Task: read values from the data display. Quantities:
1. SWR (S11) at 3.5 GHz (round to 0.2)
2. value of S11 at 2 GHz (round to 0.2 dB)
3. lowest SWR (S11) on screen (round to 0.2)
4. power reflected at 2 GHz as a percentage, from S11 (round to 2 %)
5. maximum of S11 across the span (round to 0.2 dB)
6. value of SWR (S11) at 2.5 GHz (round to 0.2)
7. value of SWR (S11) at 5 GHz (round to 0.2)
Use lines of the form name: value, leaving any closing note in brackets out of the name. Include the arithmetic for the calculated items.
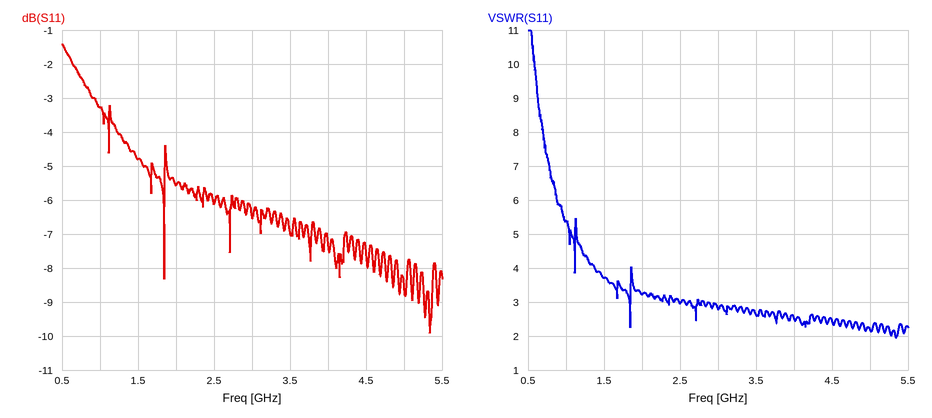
SWR (S11) at 3.5 GHz: 2.6
value of S11 at 2 GHz: -5.6 dB
lowest SWR (S11) on screen: 2.0
power reflected at 2 GHz as a percentage, from S11: 10^(-5.6/10) ≈ 28 %
maximum of S11 across the span: -1.4 dB
value of SWR (S11) at 2.5 GHz: 3.0
value of SWR (S11) at 5 GHz: 2.2
